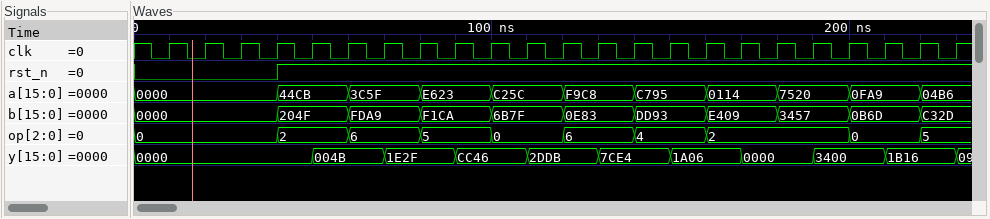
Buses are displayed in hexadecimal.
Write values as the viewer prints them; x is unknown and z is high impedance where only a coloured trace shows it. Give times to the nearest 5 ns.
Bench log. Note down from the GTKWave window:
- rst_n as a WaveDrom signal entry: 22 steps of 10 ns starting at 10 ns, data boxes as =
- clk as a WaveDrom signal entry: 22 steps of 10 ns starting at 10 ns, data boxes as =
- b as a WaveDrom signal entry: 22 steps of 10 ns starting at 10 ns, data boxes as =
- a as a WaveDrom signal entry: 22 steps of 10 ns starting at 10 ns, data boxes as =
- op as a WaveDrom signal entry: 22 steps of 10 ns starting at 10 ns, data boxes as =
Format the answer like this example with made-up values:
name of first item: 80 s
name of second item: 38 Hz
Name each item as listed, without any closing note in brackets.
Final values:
rst_n as a WaveDrom signal entry: 22 steps of 10 ns starting at 10 ns, data boxes as =: {name: 'rst_n', wave: '0..1..................'}
clk as a WaveDrom signal entry: 22 steps of 10 ns starting at 10 ns, data boxes as =: {name: 'clk', wave: 'p.....................'}
b as a WaveDrom signal entry: 22 steps of 10 ns starting at 10 ns, data boxes as =: {name: 'b', wave: '=..=.=.=.=.=.=.=.=.=.=', data: '0000 204F FDA9 F1CA 6B7F 0E83 DD93 E409 3457 0B6D C32D'}
a as a WaveDrom signal entry: 22 steps of 10 ns starting at 10 ns, data boxes as =: {name: 'a', wave: '=..=.=.=.=.=.=.=.=.=.=', data: '0000 44CB 3C5F E623 C25C F9C8 C795 0114 7520 0FA9 04B6'}
op as a WaveDrom signal entry: 22 steps of 10 ns starting at 10 ns, data boxes as =: {name: 'op', wave: '=..=.=.=.=.=.=.=...=.=', data: '0 2 6 5 0 6 4 2 0 5'}
